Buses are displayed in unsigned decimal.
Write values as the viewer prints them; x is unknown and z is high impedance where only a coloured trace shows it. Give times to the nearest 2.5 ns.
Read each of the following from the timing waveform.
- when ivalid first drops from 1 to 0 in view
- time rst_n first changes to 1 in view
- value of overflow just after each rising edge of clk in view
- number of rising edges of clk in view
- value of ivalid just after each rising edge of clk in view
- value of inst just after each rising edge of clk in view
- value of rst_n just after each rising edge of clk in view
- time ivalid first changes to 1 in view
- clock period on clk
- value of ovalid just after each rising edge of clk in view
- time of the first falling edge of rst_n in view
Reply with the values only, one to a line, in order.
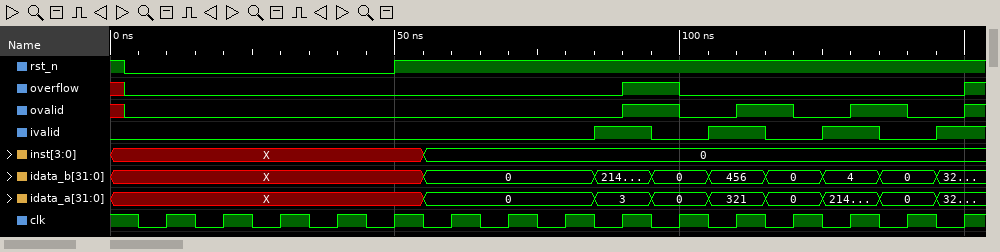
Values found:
95 ns
50 ns
0 0 0 0 0 0 0 0 1 0 0 0 0 0 1
15
0 0 0 0 0 0 0 0 1 0 1 0 1 0 1
X, X, X, X, X, 0, 0, 0, 0, 0, 0, 0, 0, 0, 0
0 0 0 0 1 1 1 1 1 1 1 1 1 1 1
85 ns
10 ns
0 0 0 0 0 0 0 0 1 0 1 0 1 0 1
2.5 ns
